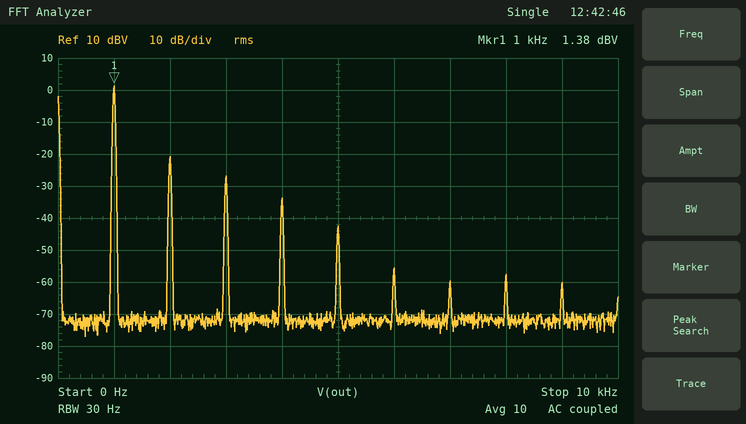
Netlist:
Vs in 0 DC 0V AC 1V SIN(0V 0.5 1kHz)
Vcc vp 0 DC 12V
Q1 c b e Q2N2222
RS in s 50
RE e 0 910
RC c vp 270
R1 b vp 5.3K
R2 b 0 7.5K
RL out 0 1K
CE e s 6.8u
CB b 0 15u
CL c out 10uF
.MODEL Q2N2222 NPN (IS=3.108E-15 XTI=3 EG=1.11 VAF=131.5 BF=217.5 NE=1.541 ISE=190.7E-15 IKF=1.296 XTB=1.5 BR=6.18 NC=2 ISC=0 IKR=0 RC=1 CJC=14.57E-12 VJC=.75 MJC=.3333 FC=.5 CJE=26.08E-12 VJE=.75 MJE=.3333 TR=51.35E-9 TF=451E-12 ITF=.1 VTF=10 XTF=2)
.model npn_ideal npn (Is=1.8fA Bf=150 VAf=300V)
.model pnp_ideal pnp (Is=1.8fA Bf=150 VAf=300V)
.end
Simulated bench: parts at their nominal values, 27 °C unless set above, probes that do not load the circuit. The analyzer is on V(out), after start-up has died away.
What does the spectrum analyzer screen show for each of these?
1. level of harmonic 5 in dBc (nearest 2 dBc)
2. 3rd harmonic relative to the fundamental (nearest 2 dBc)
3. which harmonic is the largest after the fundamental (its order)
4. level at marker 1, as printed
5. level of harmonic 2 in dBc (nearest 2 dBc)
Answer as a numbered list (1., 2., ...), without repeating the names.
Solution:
1. -44 dBc
2. -28 dBc
3. 2
4. 1.38 dBV
5. -22 dBc
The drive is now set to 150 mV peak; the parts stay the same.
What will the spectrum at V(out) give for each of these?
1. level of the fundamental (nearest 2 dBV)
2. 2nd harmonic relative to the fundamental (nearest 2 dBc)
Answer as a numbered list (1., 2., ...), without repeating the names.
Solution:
1. -8 dBV
2. -42 dBc
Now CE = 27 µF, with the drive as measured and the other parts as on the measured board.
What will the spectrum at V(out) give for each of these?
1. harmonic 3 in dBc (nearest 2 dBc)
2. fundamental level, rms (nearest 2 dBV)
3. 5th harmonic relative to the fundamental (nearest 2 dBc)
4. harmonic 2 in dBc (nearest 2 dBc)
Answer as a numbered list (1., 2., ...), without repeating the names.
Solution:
1. -26 dBc
2. 2 dBV
3. -46 dBc
4. -20 dBc
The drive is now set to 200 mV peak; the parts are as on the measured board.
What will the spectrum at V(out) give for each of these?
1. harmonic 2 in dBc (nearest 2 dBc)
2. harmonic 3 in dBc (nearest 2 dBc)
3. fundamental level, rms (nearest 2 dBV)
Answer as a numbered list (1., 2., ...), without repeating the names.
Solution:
1. -40 dBc
2. -56 dBc
3. -6 dBV
